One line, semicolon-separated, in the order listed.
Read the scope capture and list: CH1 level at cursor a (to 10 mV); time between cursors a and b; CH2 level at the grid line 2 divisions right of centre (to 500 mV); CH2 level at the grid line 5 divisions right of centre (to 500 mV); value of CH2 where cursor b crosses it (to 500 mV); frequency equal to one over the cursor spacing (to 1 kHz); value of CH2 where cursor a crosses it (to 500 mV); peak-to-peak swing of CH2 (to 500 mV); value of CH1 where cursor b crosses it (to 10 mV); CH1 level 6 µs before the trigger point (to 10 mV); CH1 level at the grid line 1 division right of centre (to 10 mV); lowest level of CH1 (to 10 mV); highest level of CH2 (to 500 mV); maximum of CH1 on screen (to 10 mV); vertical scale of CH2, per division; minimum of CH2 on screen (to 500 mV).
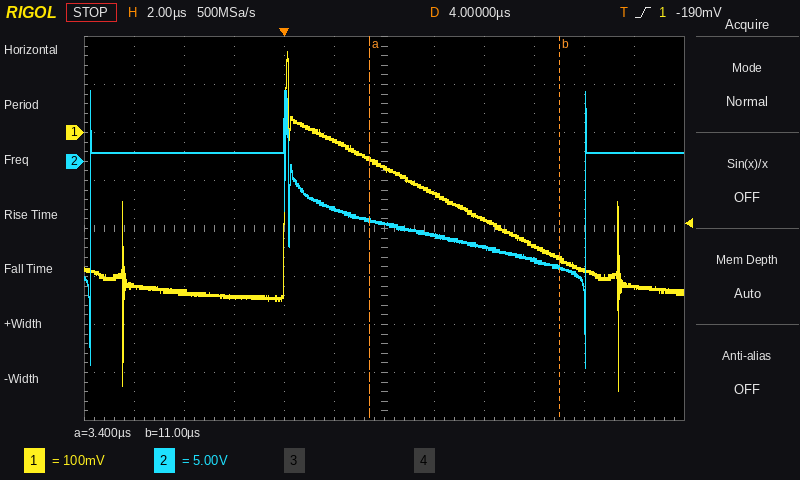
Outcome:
-60 mV; 7.6 µs; -9.0 V; 1.0 V; -11.0 V; 132 kHz; -6.0 V; 29.0 V; -260 mV; -320 mV; -130 mV; -540 mV; 7.5 V; 170 mV; 5 V; -21.5 V
